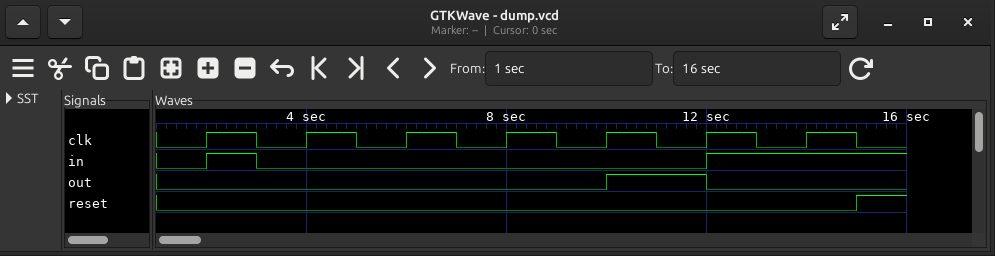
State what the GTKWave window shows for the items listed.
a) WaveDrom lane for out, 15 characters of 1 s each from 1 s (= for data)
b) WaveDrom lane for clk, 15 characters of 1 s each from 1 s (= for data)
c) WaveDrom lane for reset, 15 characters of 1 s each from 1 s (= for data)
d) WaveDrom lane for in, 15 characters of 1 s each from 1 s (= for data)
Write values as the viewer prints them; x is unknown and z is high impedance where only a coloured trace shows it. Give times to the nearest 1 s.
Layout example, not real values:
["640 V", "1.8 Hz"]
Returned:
["{name: 'out', wave: '0........1.0...'}", "{name: 'clk', wave: '010101010101010'}", "{name: 'reset', wave: '0.............1'}", "{name: 'in', wave: '010........1...'}"]
